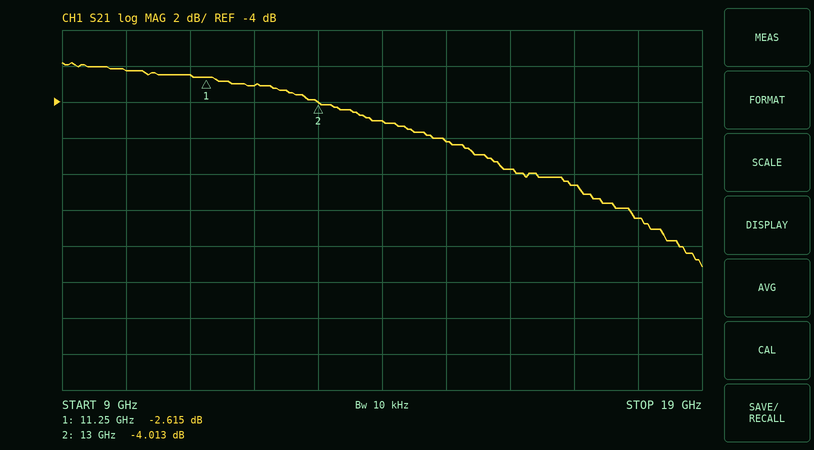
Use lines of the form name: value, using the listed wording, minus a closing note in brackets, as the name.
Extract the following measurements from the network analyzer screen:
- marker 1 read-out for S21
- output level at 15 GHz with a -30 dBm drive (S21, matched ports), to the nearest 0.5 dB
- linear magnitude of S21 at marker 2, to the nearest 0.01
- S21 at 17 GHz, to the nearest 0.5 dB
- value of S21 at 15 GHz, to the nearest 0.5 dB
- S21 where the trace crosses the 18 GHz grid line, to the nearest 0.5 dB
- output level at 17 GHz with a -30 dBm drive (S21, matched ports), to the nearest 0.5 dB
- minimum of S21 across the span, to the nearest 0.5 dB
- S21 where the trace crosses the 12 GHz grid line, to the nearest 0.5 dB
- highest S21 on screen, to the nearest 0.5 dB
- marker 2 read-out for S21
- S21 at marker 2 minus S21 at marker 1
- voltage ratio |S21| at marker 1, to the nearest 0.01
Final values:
marker 1 read-out for S21: -2.615 dB
output level at 15 GHz with a -30 dBm drive (S21, matched ports), to the nearest 0.5 dB: -36.0 dBm
linear magnitude of S21 at marker 2, to the nearest 0.01: 0.63
S21 at 17 GHz, to the nearest 0.5 dB: -8.5 dB
value of S21 at 15 GHz, to the nearest 0.5 dB: -6.0 dB
S21 where the trace crosses the 18 GHz grid line, to the nearest 0.5 dB: -10.5 dB
output level at 17 GHz with a -30 dBm drive (S21, matched ports), to the nearest 0.5 dB: -38.5 dBm
minimum of S21 across the span, to the nearest 0.5 dB: -13.0 dB
S21 where the trace crosses the 12 GHz grid line, to the nearest 0.5 dB: -3.0 dB
highest S21 on screen, to the nearest 0.5 dB: -2.0 dB
marker 2 read-out for S21: -4.013 dB
S21 at marker 2 minus S21 at marker 1: -1.398 dB
voltage ratio |S21| at marker 1, to the nearest 0.01: 0.74
